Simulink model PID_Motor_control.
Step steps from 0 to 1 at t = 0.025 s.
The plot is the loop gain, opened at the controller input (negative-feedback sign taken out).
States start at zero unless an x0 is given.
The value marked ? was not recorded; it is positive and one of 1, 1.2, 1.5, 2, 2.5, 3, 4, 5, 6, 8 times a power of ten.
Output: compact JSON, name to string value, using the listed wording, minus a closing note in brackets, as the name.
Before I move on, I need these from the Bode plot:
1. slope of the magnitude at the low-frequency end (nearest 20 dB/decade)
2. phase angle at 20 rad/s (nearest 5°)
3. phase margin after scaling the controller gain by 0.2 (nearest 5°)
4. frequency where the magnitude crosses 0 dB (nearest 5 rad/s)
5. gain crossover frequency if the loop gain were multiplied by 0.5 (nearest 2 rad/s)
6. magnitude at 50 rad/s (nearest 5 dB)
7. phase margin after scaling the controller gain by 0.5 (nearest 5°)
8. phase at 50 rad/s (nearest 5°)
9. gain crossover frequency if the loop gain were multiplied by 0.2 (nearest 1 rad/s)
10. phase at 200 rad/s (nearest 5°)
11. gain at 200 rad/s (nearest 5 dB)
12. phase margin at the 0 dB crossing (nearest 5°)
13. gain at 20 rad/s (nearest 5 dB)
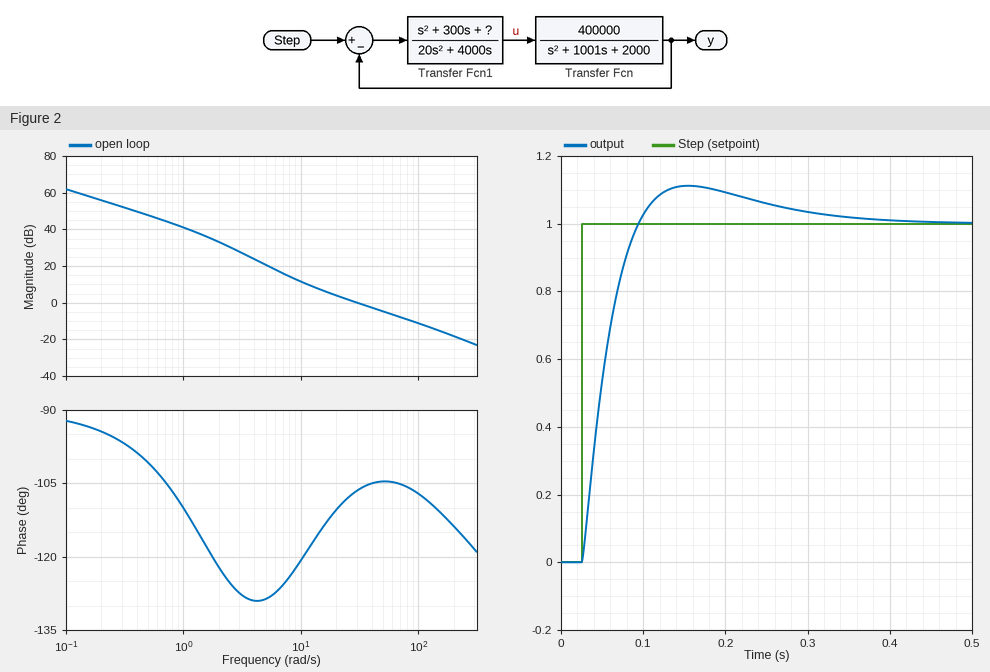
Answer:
{"slope of the magnitude at the low-frequency end": "-20 dB/decade", "phase angle at 20 rad/s": "-110°", "phase margin after scaling the controller gain by 0.2": "55°", "frequency where the magnitude crosses 0 dB": "30 rad/s", "gain crossover frequency if the loop gain were multiplied by 0.5": "16 rad/s", "magnitude at 50 rad/s": "-5 dB", "phase margin after scaling the controller gain by 0.5": "65°", "phase at 50 rad/s": "-105°", "gain crossover frequency if the loop gain were multiplied by 0.2": "8 rad/s", "phase at 200 rad/s": "-115°", "gain at 200 rad/s": "-20 dB", "phase margin at the 0 dB crossing": "75°", "gain at 20 rad/s": "5 dB"}
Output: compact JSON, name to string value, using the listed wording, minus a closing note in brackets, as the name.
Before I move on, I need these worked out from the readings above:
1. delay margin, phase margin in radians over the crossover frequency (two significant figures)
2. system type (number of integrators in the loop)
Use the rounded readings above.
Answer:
{"delay margin, phase margin in radians over the crossover frequency": "0.044 s", "system type": "1"}
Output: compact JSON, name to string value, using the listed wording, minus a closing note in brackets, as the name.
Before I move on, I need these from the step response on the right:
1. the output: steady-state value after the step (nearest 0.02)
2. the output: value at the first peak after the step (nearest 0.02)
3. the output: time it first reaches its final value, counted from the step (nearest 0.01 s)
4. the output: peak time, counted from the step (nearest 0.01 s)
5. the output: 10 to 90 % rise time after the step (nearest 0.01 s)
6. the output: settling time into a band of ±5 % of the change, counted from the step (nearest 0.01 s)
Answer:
{"the output: steady-state value after the step": "1.00", "the output: value at the first peak after the step": "1.12", "the output: time it first reaches its final value, counted from the step": "0.07 s", "the output: peak time, counted from the step": "0.13 s", "the output: 10 to 90 % rise time after the step": "0.05 s", "the output: settling time into a band of ±5 % of the change, counted from the step": "0.24 s"}
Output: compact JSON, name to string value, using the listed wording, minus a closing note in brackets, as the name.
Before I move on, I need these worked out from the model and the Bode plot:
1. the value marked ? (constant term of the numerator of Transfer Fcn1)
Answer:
{"the value marked ?": "2500"}
